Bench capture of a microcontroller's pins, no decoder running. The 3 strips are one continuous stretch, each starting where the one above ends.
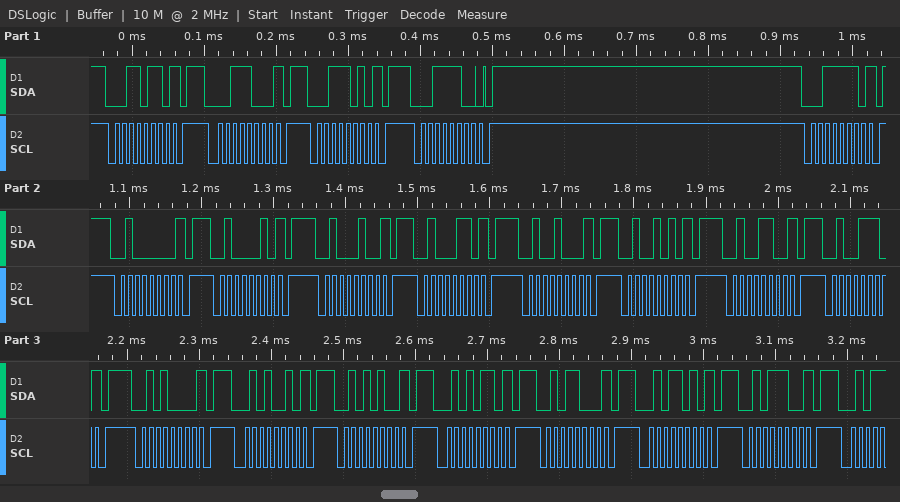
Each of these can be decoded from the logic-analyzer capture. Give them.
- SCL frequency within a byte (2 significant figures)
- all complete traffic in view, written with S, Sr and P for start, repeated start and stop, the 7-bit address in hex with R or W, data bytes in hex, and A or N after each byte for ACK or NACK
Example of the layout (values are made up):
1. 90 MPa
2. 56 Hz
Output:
1. 100 kHz
2. S 1BW N P S 1CW N P S 1DW N P S 1EW A P S 1FW N P S 20W N P S 21W N P S 22W N P S 23W N P S 24W N P S 25W N P S 26W N P S 27W N P S 28W N P S 29W N P S 2AW N P S 2BW N P S 2CW N P S 2DW N P S 2EW N P
